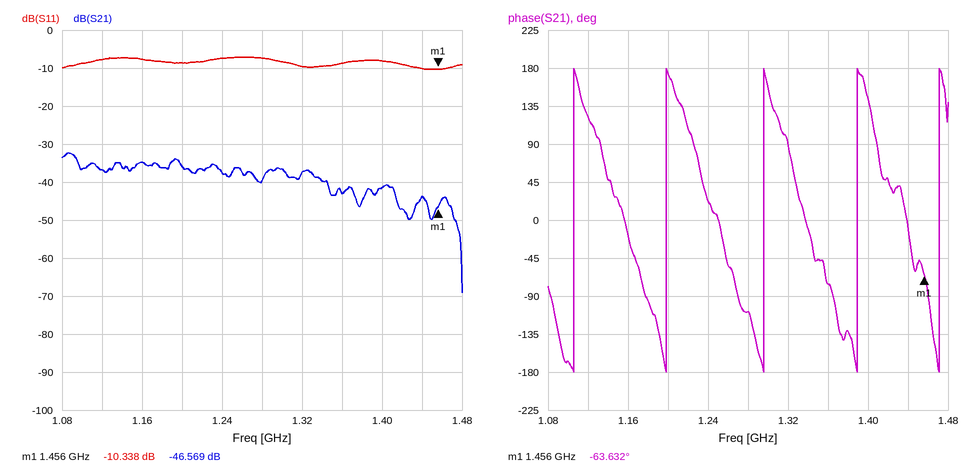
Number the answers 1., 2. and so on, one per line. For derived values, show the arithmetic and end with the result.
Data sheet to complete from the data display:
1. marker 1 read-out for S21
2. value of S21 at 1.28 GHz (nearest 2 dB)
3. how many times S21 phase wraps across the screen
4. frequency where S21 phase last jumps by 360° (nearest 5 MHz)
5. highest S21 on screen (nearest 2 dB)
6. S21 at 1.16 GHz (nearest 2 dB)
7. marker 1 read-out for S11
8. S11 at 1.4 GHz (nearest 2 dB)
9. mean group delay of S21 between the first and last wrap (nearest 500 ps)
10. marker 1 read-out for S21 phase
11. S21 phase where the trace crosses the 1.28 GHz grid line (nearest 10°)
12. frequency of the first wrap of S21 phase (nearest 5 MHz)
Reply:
1. -46.569 dB
2. -40 dB
3. 5
4. 1.470 GHz
5. -32 dB
6. -34 dB
7. -10.338 dB
8. -8 dB
9. 4 cycles / (1.470 GHz − 1.105 GHz) ≈ 11.0 ns
10. -63.632°
11. -110°
12. 1.105 GHz
